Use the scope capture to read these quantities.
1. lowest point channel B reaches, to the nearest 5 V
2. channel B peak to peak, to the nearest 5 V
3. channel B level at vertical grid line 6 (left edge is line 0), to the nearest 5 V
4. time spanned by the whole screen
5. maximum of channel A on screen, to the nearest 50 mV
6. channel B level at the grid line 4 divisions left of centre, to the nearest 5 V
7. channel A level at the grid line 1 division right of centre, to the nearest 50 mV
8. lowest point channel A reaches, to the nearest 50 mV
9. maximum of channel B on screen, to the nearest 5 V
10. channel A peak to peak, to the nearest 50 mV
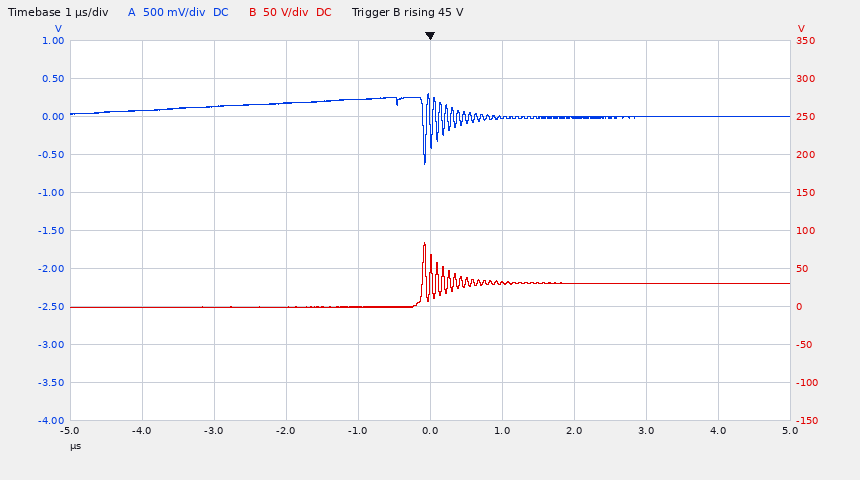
0 V
85 V
30 V
10 µs
300 mV
0 V
0 mV
-650 mV
85 V
950 mV
